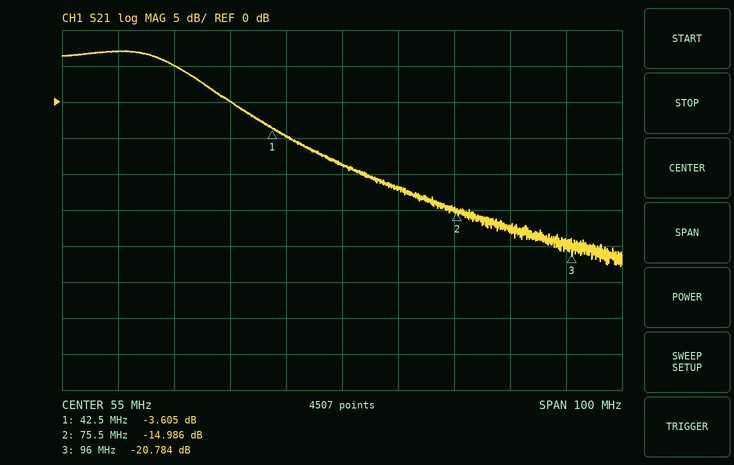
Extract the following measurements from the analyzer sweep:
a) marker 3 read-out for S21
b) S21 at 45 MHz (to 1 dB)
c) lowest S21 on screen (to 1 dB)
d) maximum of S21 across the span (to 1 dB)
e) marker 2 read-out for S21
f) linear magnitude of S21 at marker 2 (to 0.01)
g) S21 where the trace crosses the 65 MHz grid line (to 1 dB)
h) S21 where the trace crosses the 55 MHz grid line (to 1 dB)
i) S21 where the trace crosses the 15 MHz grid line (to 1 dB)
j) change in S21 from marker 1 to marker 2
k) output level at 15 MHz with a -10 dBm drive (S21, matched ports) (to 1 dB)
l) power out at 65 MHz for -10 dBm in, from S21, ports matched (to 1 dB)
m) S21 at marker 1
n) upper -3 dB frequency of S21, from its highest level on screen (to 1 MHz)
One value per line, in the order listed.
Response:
-20.784 dB
-5 dB
-23 dB
7 dB
-14.986 dB
0.18
-12 dB
-9 dB
7 dB
-11.381 dB
-3 dBm
-22 dBm
-3.605 dB
27 MHz
